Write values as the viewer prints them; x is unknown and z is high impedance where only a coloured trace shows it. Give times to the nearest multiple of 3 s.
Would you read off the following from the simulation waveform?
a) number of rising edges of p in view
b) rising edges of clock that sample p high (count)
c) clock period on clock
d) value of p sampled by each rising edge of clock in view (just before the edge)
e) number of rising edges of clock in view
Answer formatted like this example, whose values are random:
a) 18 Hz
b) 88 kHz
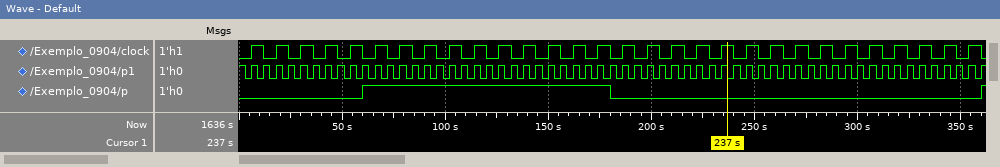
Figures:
a) 2
b) 10
c) 12 s
d) 0 0 0 0 0 1 1 1 1 1 1 1 1 1 1 0 0 0 0 0 0 0 0 0 0 0 0 0 0 0
e) 30
